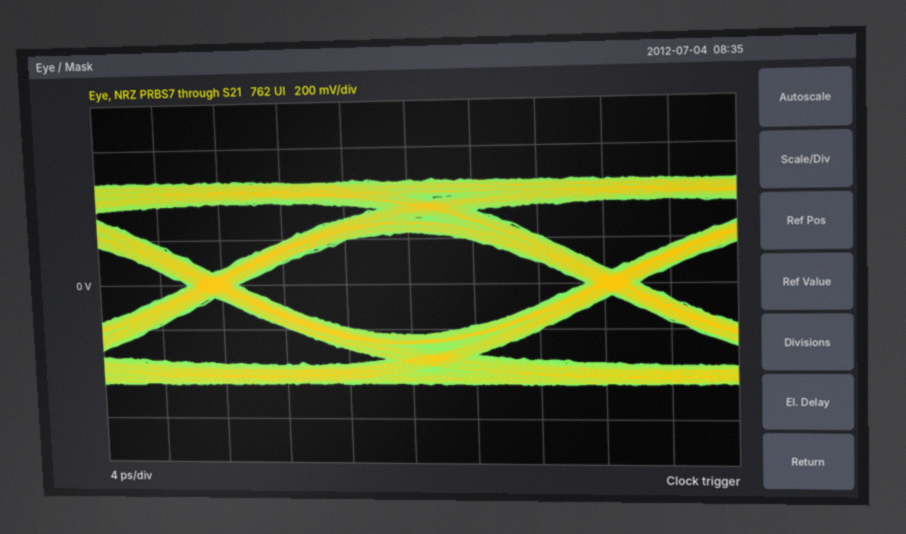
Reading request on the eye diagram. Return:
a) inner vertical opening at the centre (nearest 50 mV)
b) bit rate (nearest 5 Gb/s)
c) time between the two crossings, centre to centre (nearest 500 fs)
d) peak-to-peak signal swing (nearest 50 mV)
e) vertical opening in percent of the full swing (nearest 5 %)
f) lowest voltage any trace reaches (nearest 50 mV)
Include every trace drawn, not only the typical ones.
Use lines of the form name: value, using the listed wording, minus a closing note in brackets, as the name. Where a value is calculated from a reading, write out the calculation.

inner vertical opening at the centre: 450 mV
bit rate: 40 Gb/s
time between the two crossings, centre to centre: 25.0 ps
peak-to-peak signal swing: 900 mV
vertical opening in percent of the full swing: 450 mV / 900 mV ≈ 50 %
lowest voltage any trace reaches: -450 mV
